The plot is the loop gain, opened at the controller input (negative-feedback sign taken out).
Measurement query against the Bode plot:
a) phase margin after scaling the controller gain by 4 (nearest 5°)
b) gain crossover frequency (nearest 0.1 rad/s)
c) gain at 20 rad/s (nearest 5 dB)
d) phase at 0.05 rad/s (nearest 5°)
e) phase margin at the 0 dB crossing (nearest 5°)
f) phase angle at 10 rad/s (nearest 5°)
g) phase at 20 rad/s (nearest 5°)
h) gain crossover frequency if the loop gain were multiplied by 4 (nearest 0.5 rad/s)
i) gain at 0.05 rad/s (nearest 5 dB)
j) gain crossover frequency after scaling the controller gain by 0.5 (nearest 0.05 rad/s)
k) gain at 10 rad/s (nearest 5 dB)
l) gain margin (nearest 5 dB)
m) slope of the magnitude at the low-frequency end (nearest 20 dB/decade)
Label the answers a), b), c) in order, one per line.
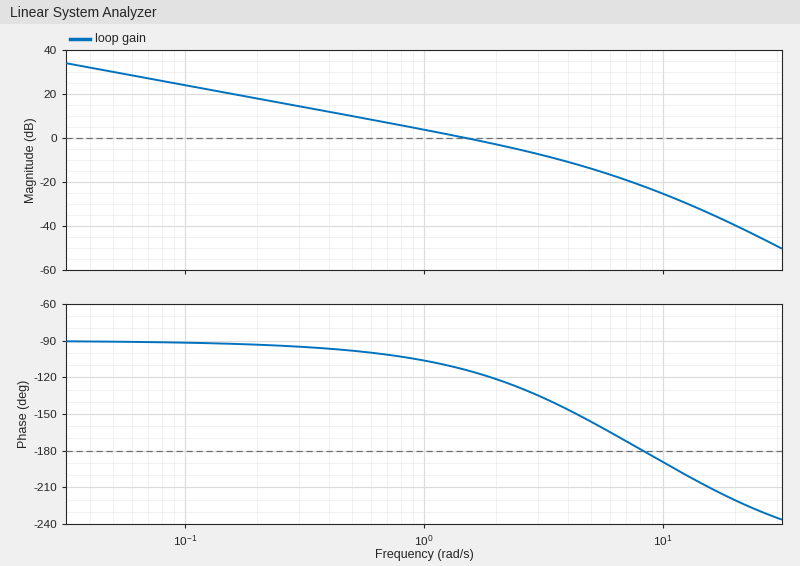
a) 30°
b) 1.5 rad/s
c) -40 dB
d) -90°
e) 65°
f) -190°
g) -220°
h) 4.5 rad/s
i) 30 dB
j) 0.80 rad/s
k) -25 dB
l) 20 dB
m) -20 dB/decade
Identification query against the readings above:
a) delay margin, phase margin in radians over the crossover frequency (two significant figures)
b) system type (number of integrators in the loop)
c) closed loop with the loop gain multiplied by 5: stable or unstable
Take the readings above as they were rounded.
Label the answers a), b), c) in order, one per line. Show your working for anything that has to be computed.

a) 65 × π / 180 / 1.5 = 0.76 s
b) 1
c) stable
